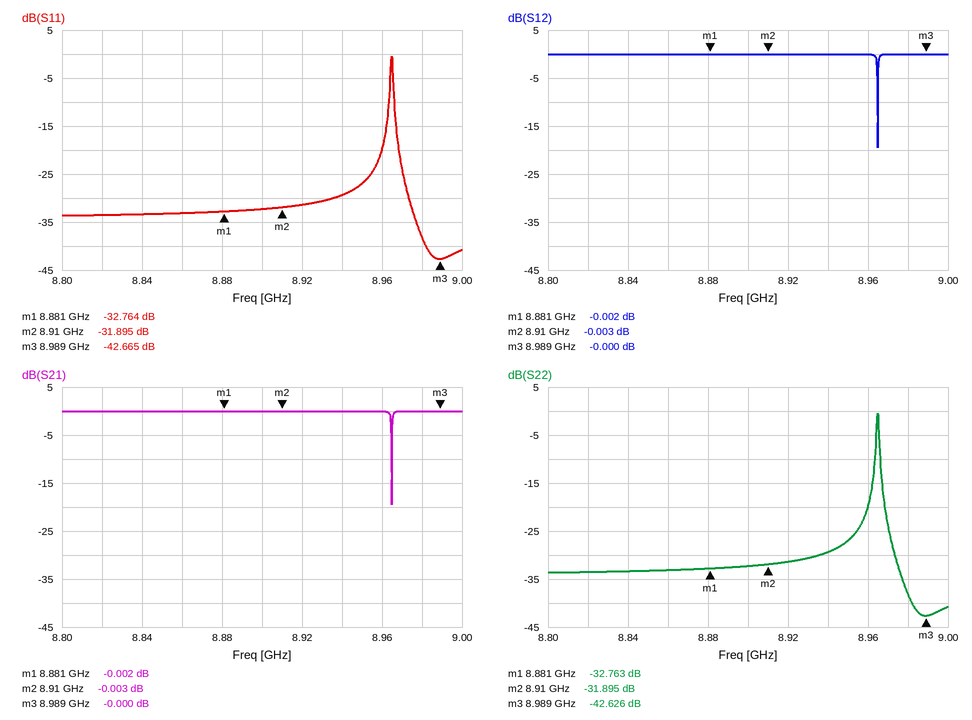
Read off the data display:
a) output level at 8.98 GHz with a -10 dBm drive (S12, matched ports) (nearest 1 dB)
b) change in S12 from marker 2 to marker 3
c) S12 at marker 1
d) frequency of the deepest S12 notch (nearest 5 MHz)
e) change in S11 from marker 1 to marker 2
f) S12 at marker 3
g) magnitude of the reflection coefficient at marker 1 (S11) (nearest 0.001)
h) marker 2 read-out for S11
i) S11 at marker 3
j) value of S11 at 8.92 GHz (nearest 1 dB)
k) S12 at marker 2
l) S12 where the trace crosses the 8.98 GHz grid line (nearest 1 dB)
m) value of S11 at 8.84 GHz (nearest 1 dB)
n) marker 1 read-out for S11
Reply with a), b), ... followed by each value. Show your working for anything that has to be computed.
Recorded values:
a) -10 dBm + (0 dB) = -10 dBm
b) -0 − (-0.003) = 0.003 dB
c) -0.002 dB
d) 8.965 GHz
e) -31.895 − (-32.764) = 0.869 dB
f) -0.000 dB
g) 10^(-32.764/20) ≈ 0.023
h) -31.895 dB
i) -42.665 dB
j) -31 dB
k) -0.003 dB
l) 0 dB
m) -33 dB
n) -32.764 dB
